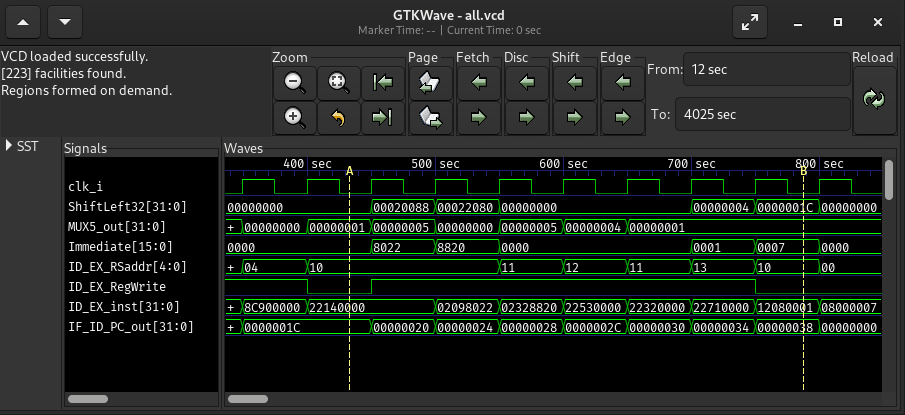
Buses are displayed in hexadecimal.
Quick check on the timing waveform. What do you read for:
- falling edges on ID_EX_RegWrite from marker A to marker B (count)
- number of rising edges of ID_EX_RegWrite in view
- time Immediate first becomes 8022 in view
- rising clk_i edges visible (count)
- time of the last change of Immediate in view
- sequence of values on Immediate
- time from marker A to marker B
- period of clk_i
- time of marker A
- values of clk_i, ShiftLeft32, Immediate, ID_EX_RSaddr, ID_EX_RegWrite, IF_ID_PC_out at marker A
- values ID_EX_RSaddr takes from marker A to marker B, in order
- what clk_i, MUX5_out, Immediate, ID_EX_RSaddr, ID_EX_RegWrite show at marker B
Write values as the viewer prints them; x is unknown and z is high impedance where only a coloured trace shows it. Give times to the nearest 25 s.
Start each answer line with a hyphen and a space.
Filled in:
- 1
- 1
- 450 s
- 10
- 800 s
- 0000, 8022, 8820, 0000, 0001, 0007, 0000
- 350 s
- 50 s
- 425 s
- clk_i=0, ShiftLeft32=00000000, Immediate=0000, ID_EX_RSaddr=10, ID_EX_RegWrite=0, IF_ID_PC_out=0000001C
- 10, 11, 12, 11, 13, 10
- clk_i=0, MUX5_out=00000001, Immediate=0007, ID_EX_RSaddr=10, ID_EX_RegWrite=0
